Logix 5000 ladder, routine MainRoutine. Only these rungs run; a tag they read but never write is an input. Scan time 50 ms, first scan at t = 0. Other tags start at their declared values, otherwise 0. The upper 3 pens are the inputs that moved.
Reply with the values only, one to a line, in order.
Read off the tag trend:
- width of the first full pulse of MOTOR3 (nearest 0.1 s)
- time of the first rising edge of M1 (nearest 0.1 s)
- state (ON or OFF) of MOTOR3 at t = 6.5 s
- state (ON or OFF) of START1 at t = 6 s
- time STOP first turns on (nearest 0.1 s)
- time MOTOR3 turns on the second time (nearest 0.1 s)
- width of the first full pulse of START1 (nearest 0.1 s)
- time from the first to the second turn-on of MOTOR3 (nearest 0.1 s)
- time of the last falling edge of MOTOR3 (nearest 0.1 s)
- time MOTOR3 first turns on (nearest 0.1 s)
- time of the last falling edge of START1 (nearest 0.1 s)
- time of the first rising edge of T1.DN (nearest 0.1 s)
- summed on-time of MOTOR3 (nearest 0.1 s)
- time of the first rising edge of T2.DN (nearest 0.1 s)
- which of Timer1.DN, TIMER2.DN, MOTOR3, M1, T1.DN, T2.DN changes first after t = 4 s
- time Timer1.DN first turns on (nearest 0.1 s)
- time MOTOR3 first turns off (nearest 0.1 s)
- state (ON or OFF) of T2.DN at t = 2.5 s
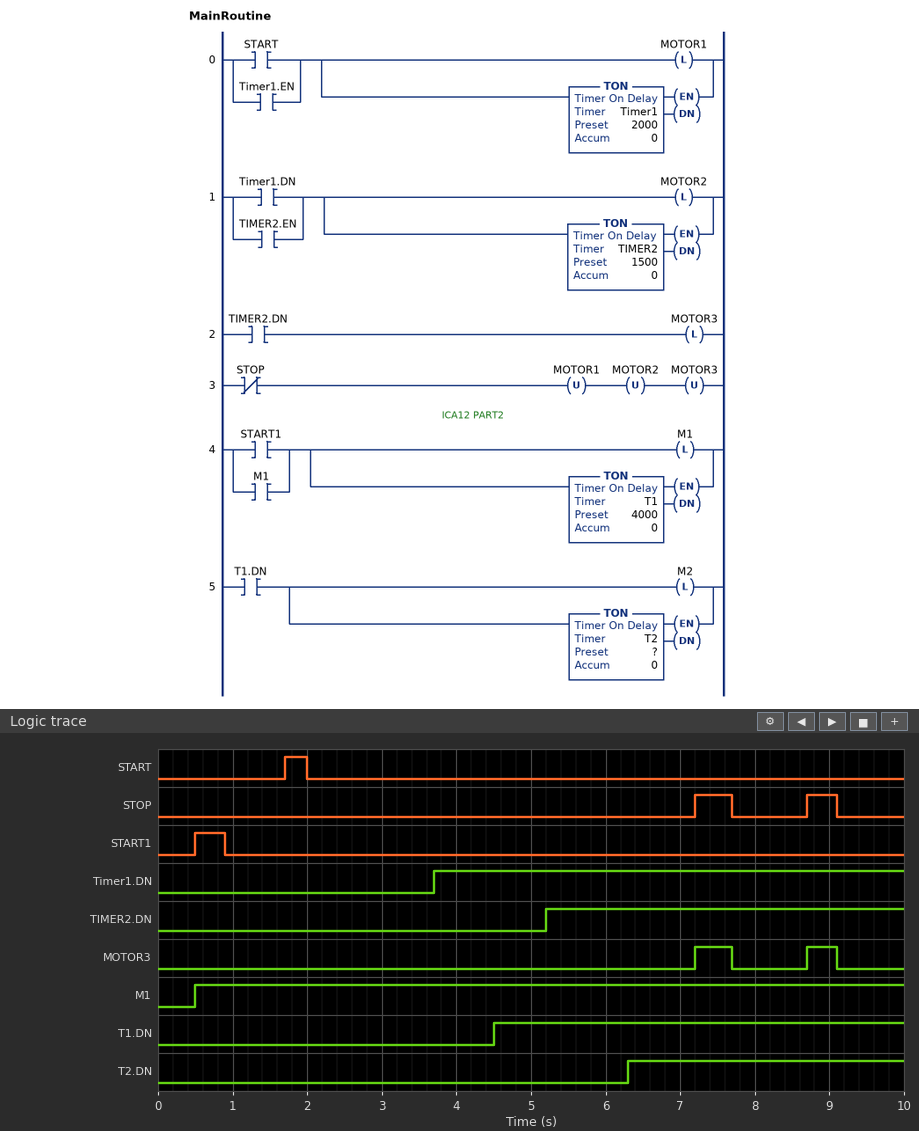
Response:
0.5 s
0.5 s
OFF
OFF
7.2 s
8.7 s
0.4 s
1.5 s
9.1 s
7.2 s
0.9 s
4.5 s
0.9 s
6.3 s
T1.DN
3.7 s
7.7 s
OFF
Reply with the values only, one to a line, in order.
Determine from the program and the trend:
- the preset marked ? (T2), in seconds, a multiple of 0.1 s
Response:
1.8 s
